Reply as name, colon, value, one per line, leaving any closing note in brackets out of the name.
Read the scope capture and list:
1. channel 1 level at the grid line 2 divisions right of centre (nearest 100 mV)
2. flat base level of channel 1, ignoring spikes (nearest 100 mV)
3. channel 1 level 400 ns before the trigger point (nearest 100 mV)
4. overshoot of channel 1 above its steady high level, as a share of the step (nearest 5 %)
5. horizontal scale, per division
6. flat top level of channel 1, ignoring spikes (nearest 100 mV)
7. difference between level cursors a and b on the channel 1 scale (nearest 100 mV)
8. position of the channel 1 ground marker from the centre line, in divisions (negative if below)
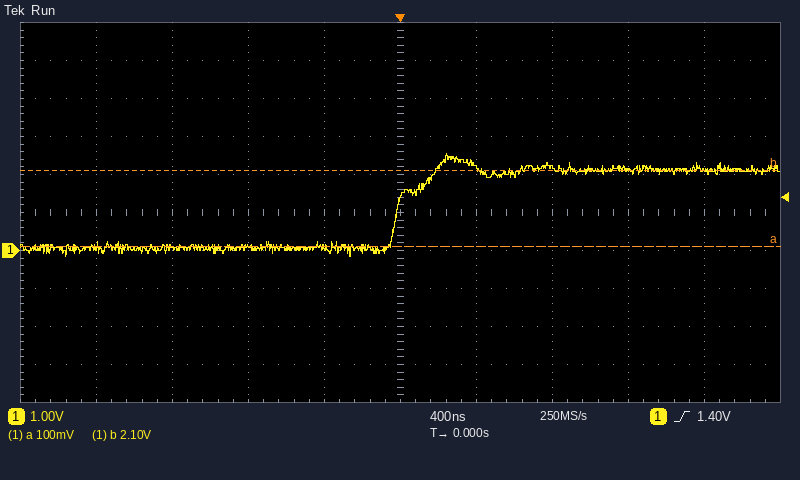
channel 1 level at the grid line 2 divisions right of centre: 2.2 V
flat base level of channel 1, ignoring spikes: 100 mV
channel 1 level 400 ns before the trigger point: 100 mV
overshoot of channel 1 above its steady high level, as a share of the step: 20 %
horizontal scale, per division: 400 ns
flat top level of channel 1, ignoring spikes: 2.1 V
difference between level cursors a and b on the channel 1 scale: 2.0 V
position of the channel 1 ground marker from the centre line, in divisions: -1.0 div
